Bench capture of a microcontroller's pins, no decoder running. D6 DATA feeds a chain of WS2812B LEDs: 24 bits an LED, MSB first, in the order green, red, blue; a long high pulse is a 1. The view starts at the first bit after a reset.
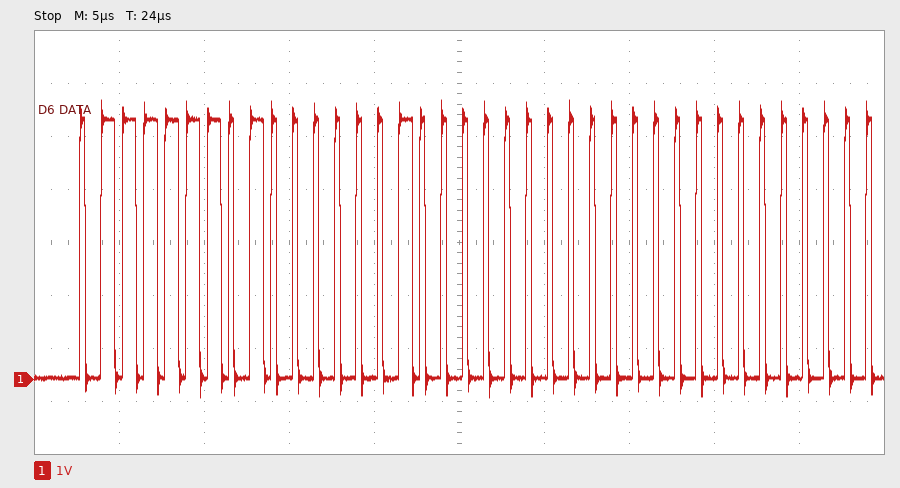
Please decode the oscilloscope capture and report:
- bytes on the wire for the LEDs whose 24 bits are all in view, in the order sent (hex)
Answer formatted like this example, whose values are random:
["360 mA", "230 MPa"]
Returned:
["7E 81 00"]
